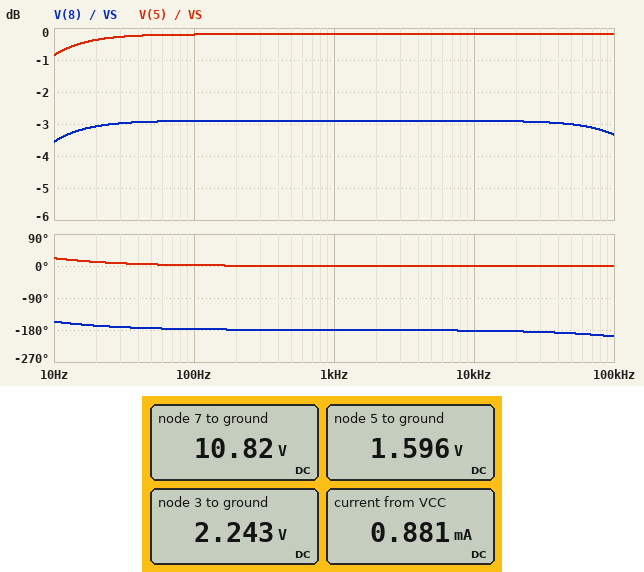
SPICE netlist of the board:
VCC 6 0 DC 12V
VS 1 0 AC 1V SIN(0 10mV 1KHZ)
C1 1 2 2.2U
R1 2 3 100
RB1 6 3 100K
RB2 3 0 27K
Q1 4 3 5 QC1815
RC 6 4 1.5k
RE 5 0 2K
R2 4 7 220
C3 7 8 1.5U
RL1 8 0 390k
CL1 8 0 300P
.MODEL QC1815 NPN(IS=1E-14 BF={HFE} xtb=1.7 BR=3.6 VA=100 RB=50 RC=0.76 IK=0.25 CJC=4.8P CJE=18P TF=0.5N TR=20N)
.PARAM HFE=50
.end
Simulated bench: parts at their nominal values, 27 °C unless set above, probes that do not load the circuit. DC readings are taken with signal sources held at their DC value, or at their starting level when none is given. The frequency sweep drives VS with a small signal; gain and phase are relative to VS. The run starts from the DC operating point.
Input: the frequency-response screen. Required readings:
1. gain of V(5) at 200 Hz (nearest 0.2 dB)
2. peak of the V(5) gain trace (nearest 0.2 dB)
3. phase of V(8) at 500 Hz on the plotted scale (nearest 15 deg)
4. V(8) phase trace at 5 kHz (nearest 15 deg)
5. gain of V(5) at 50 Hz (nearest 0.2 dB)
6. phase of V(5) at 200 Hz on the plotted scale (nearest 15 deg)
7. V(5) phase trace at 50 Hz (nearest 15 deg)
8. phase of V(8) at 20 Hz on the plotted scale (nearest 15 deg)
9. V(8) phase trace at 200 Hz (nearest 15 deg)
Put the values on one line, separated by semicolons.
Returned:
-0.2 dB; -0.2 dB; -180 deg; -180 deg; -0.2 dB; 0 deg; 0 deg; -165 deg; -180 deg
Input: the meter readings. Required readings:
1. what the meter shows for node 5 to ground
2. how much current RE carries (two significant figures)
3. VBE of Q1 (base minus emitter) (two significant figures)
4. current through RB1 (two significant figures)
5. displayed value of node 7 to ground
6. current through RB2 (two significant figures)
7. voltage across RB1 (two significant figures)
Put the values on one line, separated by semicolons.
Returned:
1.596 V; 800 µA; 650 mV; 98 µA; 10.82 V; 83 µA; 9.8 V
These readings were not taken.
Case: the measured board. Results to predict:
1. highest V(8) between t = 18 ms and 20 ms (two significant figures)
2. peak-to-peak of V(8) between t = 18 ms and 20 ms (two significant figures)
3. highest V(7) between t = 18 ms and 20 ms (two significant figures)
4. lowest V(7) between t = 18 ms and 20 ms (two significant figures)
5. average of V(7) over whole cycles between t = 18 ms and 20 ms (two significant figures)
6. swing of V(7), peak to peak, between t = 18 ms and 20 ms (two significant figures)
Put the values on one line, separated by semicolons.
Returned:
7.2 mV; 14 mV; 11 V; 11 V; 11 V; 14 mV
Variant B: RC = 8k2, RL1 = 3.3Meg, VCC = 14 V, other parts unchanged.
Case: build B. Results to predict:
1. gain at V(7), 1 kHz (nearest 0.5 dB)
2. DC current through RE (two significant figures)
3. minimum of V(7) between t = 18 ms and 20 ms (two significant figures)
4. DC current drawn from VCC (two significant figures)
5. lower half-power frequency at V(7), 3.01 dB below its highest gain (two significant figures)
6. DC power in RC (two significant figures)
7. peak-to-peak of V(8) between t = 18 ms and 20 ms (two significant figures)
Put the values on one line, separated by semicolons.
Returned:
12.0 dB; 970 µA; 6.2 V; 1.1 mA; 4.1 Hz; 7.4 mW; 78 mV
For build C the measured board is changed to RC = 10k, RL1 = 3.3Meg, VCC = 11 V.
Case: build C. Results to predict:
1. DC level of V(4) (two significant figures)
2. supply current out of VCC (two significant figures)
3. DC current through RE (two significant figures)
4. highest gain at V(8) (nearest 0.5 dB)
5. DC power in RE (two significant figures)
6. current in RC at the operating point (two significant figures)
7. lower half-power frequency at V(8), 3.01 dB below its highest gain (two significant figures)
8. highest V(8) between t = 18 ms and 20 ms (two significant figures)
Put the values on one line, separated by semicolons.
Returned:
4.1 V; 780 µA; 700 µA; 13.5 dB; 990 µW; 690 µA; 4.1 Hz; 48 mV
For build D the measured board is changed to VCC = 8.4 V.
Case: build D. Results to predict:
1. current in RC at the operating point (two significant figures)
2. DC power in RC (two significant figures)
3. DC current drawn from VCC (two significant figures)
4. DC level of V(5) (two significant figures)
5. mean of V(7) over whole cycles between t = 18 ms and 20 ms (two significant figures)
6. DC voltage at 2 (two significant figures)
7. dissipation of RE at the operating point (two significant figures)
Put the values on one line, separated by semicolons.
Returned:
470 µA; 330 µW; 540 µA; 960 mV; 7.7 V; 1.6 V; 460 µW
